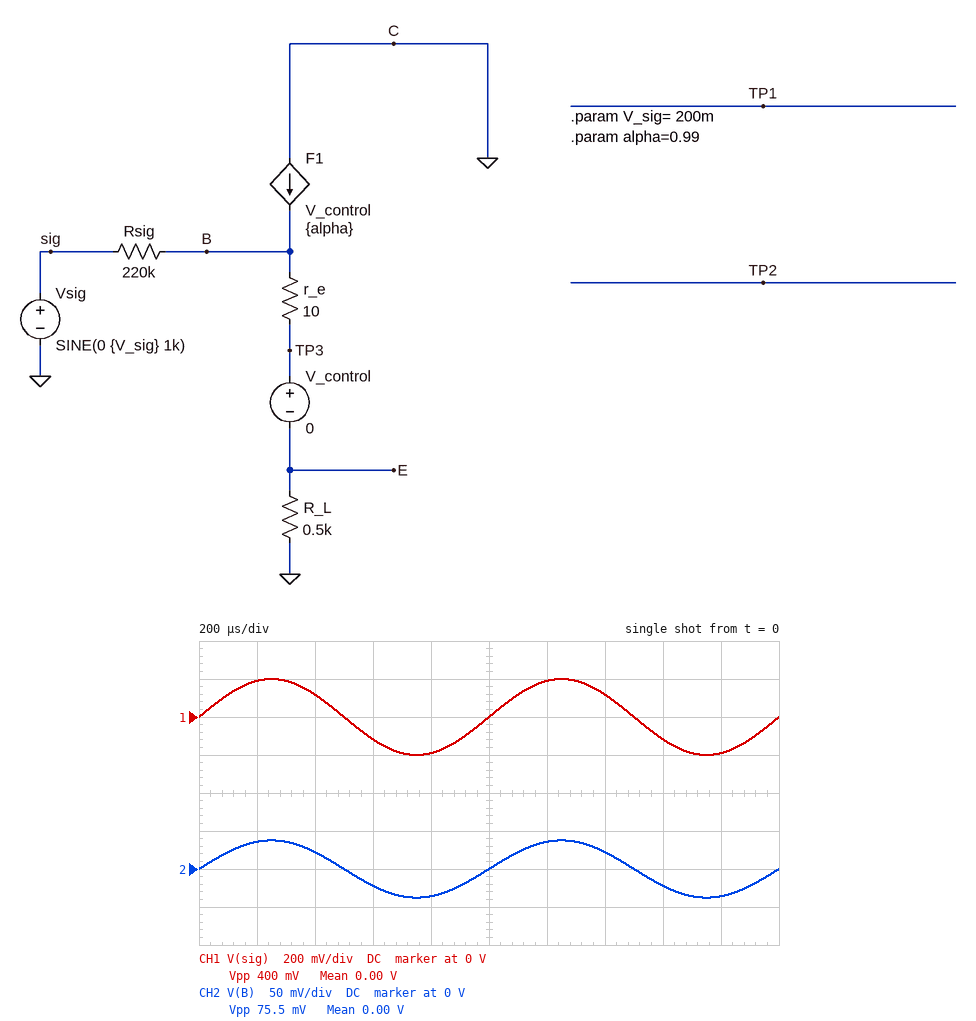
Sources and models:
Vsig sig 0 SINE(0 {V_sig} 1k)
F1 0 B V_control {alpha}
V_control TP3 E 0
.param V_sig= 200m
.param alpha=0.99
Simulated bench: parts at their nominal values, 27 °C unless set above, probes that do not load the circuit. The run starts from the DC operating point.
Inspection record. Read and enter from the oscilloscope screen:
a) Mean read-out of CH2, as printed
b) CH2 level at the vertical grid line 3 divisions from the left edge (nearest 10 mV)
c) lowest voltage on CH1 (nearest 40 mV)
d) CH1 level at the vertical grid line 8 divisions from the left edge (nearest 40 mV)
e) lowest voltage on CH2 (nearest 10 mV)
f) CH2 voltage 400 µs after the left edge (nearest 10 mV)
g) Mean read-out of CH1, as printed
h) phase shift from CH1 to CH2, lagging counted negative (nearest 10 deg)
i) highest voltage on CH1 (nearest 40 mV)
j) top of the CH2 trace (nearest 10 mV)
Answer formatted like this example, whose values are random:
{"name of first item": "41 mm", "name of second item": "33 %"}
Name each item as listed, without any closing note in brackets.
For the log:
{"Mean read-out of CH2, as printed": "0.00 V", "CH2 level at the vertical grid line 3 divisions from the left edge": "-20 mV", "lowest voltage on CH1": "-200 mV", "CH1 level at the vertical grid line 8 divisions from the left edge": "-120 mV", "lowest voltage on CH2": "-40 mV", "CH2 voltage 400 µs after the left edge": "20 mV", "Mean read-out of CH1, as printed": "0.00 V", "phase shift from CH1 to CH2, lagging counted negative": "0 deg", "highest voltage on CH1": "200 mV", "top of the CH2 trace": "40 mV"}
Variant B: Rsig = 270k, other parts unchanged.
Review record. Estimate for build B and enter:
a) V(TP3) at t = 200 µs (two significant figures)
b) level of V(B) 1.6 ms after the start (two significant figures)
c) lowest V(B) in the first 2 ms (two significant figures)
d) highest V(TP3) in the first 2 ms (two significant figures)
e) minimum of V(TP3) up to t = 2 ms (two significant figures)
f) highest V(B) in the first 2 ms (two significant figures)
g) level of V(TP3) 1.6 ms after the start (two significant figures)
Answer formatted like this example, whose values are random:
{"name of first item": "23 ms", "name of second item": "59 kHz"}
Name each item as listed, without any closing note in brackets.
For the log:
{"V(TP3) at t = 200 µs": "30 mV", "level of V(B) 1.6 ms after the start": "-19 mV", "lowest V(B) in the first 2 ms": "-32 mV", "highest V(TP3) in the first 2 ms": "31 mV", "minimum of V(TP3) up to t = 2 ms": "-31 mV", "highest V(B) in the first 2 ms": "32 mV", "level of V(TP3) 1.6 ms after the start": "-18 mV"}
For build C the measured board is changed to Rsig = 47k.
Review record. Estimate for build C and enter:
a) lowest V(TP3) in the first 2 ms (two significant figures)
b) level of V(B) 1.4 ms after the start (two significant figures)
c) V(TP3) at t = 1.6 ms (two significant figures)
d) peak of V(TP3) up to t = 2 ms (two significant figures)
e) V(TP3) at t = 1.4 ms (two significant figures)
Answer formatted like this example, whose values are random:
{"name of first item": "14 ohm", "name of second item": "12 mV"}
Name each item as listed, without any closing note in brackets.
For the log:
{"lowest V(TP3) in the first 2 ms": "-100 mV", "level of V(B) 1.4 ms after the start": "61 mV", "V(TP3) at t = 1.6 ms": "-60 mV", "peak of V(TP3) up to t = 2 ms": "100 mV", "V(TP3) at t = 1.4 ms": "60 mV"}
